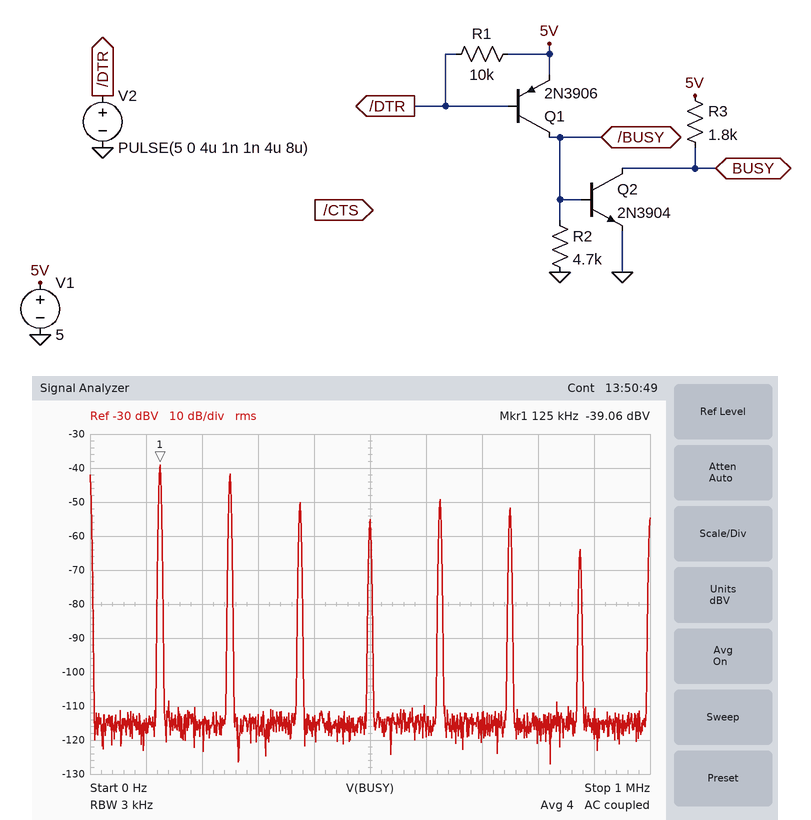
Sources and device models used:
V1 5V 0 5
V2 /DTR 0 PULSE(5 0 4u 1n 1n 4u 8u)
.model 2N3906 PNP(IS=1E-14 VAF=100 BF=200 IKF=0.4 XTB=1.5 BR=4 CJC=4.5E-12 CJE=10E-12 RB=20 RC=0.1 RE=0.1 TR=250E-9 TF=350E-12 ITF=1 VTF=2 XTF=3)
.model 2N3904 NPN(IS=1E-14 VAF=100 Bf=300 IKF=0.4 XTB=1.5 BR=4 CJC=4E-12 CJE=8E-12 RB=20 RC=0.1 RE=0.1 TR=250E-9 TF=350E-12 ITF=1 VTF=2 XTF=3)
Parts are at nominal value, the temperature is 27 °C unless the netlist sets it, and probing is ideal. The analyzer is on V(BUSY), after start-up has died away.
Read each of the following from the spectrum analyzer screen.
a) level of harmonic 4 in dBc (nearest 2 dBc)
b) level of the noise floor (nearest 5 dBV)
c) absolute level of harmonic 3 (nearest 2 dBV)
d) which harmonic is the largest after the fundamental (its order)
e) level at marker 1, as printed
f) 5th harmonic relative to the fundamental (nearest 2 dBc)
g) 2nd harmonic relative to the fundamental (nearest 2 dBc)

-16 dBc
-115 dBV
-50 dBV
2
-39.06 dBV
-10 dBc
-2 dBc
